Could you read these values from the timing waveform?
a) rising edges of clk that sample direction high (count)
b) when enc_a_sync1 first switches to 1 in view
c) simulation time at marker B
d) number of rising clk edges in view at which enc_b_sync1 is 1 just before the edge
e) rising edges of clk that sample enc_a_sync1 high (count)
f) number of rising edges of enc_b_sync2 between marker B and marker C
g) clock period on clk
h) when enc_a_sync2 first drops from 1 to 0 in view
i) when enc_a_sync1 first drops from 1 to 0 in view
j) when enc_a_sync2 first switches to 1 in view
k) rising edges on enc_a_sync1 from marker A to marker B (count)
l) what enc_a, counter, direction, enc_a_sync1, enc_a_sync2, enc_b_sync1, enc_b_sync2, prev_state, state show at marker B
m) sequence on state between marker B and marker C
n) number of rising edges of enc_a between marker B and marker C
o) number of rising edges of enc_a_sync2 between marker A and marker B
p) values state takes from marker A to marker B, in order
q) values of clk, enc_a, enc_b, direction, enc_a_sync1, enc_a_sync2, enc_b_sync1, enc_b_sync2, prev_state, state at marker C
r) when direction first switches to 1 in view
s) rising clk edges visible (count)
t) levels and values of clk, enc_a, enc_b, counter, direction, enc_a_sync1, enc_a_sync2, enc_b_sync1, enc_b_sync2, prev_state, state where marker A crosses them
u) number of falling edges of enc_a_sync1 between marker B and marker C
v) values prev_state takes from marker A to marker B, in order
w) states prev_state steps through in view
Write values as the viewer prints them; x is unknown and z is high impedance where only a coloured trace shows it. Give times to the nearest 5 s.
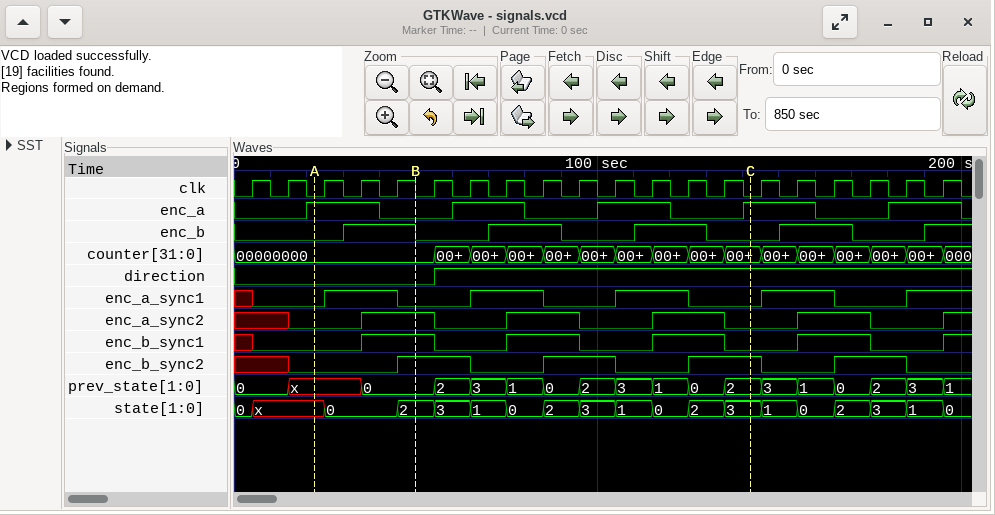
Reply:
14
25 s
50 s
8
9
2
10 s
55 s
45 s
35 s
1
enc_a=0, counter=00000000, direction=0, enc_a_sync1=0, enc_a_sync2=1, enc_b_sync1=1, enc_b_sync2=1, prev_state=0, state=2
2, 3, 1, 0, 2, 3, 1, 0, 2, 3
3
1
x, 0, 2
clk=0, enc_a=1, enc_b=0, direction=1, enc_a_sync1=0, enc_a_sync2=0, enc_b_sync1=0, enc_b_sync2=1, prev_state=2, state=3
55 s
20
clk=0, enc_a=1, enc_b=0, counter=00000000, direction=0, enc_a_sync1=0, enc_a_sync2=0, enc_b_sync1=0, enc_b_sync2=0, prev_state=x, state=x
2
x, 0
0, x, 0, 2, 3, 1, 0, 2, 3, 1, 0, 2, 3, 1, 0, 2, 3, 1
